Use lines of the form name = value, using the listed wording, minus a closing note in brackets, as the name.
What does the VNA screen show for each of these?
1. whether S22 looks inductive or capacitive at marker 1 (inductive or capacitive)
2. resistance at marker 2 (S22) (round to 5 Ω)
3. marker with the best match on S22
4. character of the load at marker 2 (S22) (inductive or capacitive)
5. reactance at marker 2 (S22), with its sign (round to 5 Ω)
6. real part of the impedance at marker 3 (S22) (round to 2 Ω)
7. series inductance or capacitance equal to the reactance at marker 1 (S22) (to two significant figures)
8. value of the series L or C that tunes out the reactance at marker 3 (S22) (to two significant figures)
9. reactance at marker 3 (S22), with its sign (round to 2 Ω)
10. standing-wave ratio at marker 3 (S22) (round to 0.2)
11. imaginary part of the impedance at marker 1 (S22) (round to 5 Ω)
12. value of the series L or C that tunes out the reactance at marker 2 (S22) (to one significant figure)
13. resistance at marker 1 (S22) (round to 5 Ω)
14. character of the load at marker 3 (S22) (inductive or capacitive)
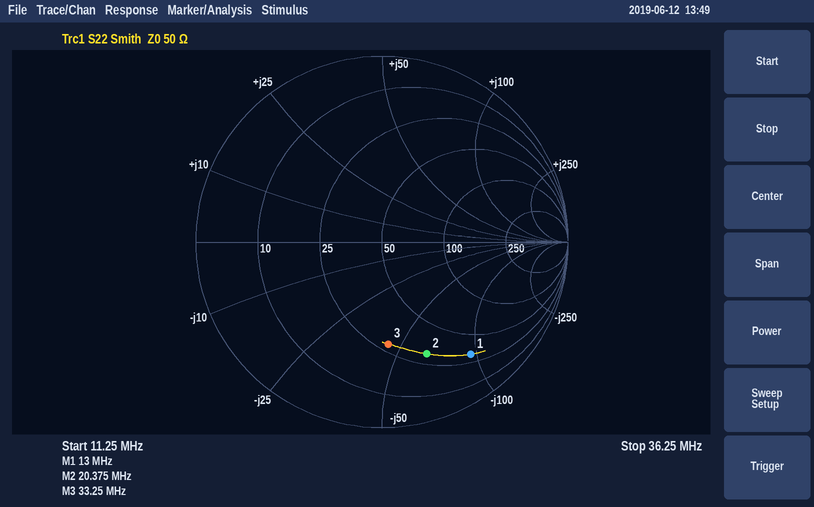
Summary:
whether S22 looks inductive or capacitive at marker 1 = capacitive
resistance at marker 2 (S22) = 30 Ω
marker with the best match on S22 = marker 3
character of the load at marker 2 (S22) = capacitive
reactance at marker 2 (S22), with its sign = -65 Ω
real part of the impedance at marker 3 (S22) = 28 Ω
series inductance or capacitance equal to the reactance at marker 1 (S22) = 130 pF
value of the series L or C that tunes out the reactance at marker 3 (S22) = 210 nH
reactance at marker 3 (S22), with its sign = -44 Ω
standing-wave ratio at marker 3 (S22) = 3.4
imaginary part of the impedance at marker 1 (S22) = -95 Ω
value of the series L or C that tunes out the reactance at marker 2 (S22) = 500 nH
resistance at marker 1 (S22) = 30 Ω
character of the load at marker 3 (S22) = capacitive
